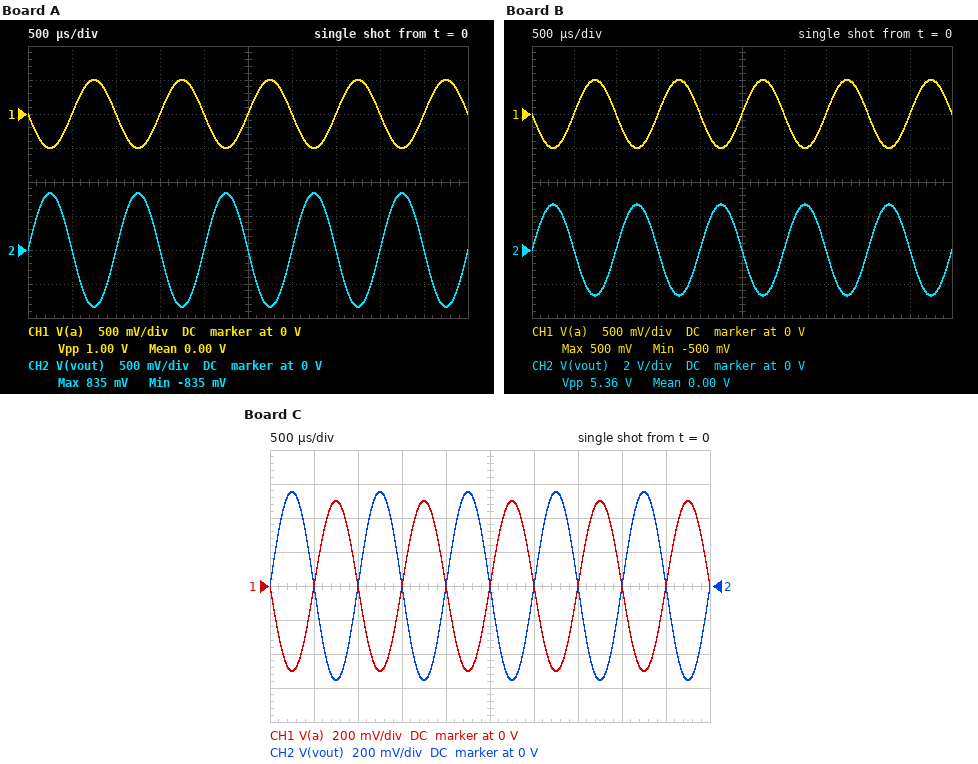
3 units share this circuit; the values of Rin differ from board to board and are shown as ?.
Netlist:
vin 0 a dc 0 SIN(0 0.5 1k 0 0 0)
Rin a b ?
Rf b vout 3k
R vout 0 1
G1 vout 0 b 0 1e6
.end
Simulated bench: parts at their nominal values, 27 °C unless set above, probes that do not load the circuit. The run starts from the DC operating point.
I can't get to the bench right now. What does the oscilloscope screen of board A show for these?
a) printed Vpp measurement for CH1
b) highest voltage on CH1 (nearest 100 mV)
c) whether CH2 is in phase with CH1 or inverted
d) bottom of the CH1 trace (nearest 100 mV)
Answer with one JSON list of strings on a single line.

["1.00 V", "500 mV", "inverted", "-500 mV"]
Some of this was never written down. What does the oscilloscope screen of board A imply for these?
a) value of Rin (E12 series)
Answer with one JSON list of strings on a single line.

["1.8 kΩ"]
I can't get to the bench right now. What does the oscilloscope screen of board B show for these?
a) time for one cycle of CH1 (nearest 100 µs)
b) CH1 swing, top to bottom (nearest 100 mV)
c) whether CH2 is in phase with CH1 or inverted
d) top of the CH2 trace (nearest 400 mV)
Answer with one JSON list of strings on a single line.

["1.0 ms", "1.0 V", "inverted", "2.8 V"]
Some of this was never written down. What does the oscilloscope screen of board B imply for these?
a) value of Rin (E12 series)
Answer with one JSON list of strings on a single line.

["560 Ω"]
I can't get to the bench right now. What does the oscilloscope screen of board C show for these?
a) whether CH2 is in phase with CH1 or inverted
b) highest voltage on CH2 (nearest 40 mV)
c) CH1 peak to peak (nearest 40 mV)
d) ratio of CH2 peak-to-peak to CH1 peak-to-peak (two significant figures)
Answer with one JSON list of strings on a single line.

["inverted", "560 mV", "1.00 V", "1.1"]
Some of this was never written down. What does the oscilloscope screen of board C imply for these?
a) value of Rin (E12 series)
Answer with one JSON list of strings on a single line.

["2.7 kΩ"]
